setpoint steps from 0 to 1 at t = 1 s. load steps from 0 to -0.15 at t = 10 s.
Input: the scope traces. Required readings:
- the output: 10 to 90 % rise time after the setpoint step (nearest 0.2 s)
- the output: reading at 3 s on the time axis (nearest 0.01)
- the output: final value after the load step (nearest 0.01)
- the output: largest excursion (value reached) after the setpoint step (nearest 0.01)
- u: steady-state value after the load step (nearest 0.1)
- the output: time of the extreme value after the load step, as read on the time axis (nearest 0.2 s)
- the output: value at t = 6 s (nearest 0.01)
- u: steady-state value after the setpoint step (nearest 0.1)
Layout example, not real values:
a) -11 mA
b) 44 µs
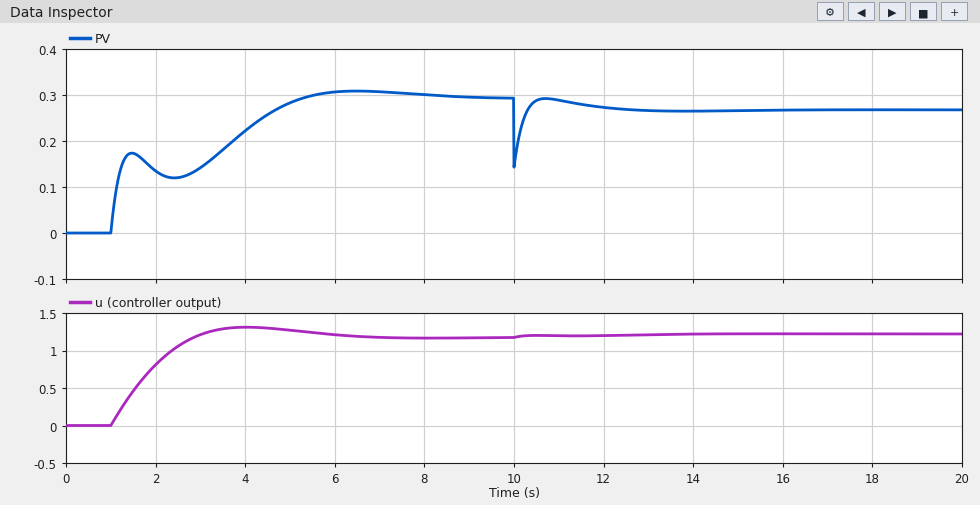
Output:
a) 3.6 s
b) 0.14
c) 0.27
d) 0.31
e) 1.2
f) 10.0 s
g) 0.31
h) 1.2
